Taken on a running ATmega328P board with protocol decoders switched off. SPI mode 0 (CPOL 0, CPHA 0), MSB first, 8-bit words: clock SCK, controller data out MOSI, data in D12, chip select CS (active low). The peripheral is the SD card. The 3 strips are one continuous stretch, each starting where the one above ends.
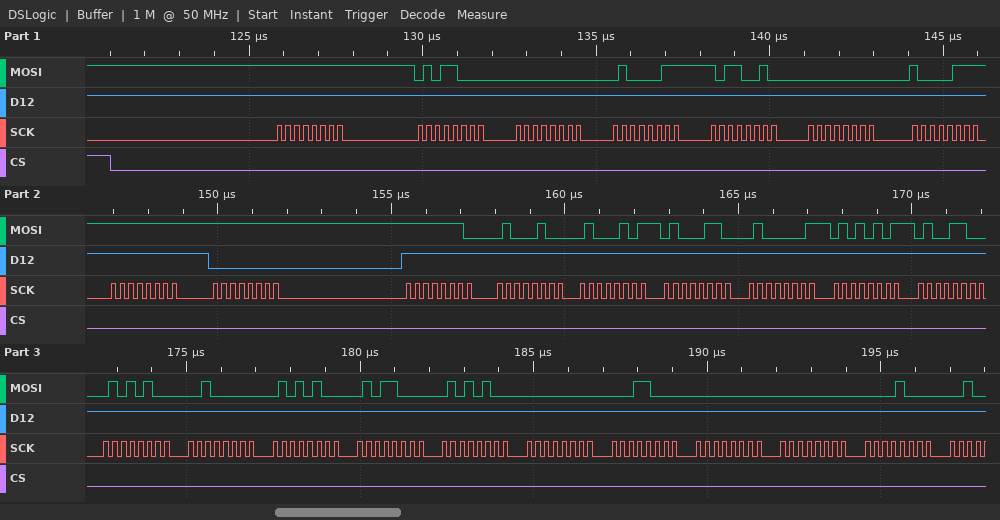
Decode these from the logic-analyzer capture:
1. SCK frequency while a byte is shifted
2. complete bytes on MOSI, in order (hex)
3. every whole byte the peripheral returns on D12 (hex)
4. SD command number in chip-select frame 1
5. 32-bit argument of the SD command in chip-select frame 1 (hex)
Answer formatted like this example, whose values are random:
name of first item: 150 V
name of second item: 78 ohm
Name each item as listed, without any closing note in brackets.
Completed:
SCK frequency while a byte is shifted: 4 MHz
complete bytes on MOSI, in order: FF 58 00 43 B2 00 87 FF FF FE 44 45 46 41 55 4C 54 20 54 58 54 00 18 00 00 08
every whole byte the peripheral returns on D12: FF FF FF FF FF FF FF FF 00 FF FF FF FF FF FF FF FF FF FF FF FF FF FF FF FF FF
SD command number in chip-select frame 1: CMD24
32-bit argument of the SD command in chip-select frame 1: 0x0043B200
